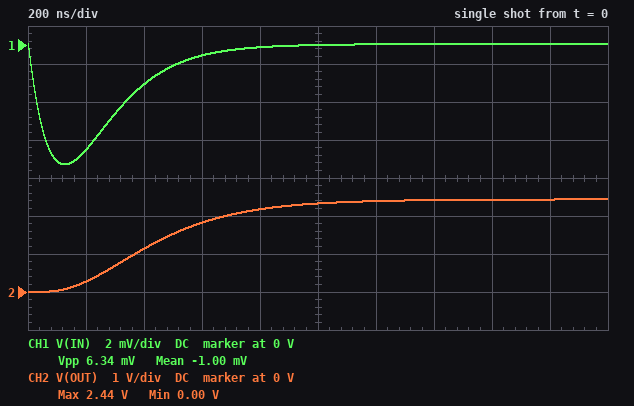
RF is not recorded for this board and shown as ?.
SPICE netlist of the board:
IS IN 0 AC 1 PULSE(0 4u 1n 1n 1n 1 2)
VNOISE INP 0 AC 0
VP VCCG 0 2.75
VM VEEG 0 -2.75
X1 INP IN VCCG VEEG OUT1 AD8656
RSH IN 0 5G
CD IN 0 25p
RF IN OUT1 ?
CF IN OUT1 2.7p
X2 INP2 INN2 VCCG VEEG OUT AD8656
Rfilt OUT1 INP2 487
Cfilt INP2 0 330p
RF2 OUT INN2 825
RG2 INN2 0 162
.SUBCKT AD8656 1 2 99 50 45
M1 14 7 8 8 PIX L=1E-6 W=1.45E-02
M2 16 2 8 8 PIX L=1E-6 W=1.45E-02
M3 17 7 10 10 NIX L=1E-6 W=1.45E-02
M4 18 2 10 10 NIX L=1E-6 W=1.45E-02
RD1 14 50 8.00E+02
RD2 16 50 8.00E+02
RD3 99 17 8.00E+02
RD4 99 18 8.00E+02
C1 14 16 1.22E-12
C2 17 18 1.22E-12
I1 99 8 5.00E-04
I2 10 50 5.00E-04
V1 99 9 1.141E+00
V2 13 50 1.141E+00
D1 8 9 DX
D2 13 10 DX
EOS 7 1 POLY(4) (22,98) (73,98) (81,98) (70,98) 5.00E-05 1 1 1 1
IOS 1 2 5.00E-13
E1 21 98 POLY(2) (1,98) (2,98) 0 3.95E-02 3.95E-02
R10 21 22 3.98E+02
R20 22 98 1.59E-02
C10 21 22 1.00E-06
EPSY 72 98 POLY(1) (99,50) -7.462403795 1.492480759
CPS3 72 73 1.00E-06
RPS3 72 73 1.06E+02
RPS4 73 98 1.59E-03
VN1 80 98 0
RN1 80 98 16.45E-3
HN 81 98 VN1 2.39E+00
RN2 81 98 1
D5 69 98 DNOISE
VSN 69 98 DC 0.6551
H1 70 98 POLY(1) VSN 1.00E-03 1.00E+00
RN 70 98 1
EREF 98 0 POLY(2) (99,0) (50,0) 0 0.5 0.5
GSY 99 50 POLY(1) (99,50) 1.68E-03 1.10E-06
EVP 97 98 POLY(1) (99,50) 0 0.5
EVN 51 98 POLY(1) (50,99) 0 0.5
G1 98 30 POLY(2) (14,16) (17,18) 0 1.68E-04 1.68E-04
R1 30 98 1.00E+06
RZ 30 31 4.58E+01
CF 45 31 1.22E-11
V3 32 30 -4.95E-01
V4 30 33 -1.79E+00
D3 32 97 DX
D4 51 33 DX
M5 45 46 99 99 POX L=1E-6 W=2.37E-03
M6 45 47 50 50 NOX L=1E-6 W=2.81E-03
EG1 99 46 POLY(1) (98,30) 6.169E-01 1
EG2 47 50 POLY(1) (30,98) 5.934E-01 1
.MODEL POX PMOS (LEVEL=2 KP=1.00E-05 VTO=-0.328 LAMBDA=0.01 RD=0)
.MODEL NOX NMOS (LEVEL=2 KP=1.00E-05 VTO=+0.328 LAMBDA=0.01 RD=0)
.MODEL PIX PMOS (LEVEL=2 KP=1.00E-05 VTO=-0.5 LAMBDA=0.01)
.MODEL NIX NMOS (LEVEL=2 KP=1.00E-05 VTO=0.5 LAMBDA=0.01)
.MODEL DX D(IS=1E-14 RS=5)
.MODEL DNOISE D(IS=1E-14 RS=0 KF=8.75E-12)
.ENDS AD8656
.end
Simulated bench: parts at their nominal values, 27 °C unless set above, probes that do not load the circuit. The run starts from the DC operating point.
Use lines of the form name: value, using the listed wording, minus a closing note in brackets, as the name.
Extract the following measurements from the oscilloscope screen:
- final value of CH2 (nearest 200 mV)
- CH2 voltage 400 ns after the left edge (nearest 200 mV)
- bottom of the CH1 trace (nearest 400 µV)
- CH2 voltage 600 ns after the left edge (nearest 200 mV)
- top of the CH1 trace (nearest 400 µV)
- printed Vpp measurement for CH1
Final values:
final value of CH2: 2.4 V
CH2 voltage 400 ns after the left edge: 1.2 V
bottom of the CH1 trace: -6.4 mV
CH2 voltage 600 ns after the left edge: 1.8 V
top of the CH1 trace: 0 V
printed Vpp measurement for CH1: 6.34 mV
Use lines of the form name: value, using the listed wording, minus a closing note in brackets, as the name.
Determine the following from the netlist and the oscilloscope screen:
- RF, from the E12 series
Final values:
RF, from the E12 series: 100 kΩ
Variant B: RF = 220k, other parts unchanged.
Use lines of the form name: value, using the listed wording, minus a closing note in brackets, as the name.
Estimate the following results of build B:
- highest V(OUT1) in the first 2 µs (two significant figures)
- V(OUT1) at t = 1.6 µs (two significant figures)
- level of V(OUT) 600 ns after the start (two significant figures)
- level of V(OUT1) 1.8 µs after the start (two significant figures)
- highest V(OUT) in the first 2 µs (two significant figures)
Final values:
highest V(OUT1) in the first 2 µs: 860 mV
V(OUT1) at t = 1.6 µs: 830 mV
level of V(OUT) 600 ns after the start: 2.4 V
level of V(OUT1) 1.8 µs after the start: 850 mV
highest V(OUT) in the first 2 µs: 2.7 V
